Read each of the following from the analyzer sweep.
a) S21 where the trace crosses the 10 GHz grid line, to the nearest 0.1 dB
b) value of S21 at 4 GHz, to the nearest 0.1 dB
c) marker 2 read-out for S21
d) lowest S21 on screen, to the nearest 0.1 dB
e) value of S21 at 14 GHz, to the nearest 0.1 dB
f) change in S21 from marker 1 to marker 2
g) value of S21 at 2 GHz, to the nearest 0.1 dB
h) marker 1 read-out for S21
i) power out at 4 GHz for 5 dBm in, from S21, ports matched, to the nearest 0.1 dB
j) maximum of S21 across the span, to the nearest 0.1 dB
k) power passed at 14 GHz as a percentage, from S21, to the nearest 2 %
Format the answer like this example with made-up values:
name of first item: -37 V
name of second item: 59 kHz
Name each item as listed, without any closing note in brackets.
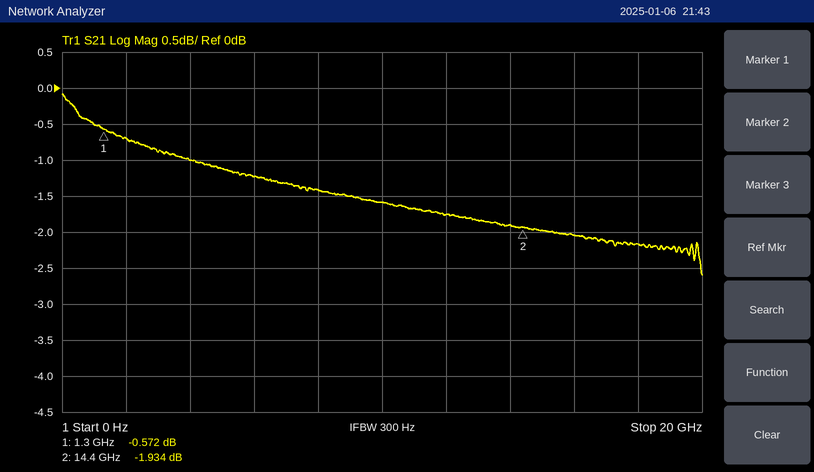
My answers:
S21 where the trace crosses the 10 GHz grid line, to the nearest 0.1 dB: -1.6 dB
value of S21 at 4 GHz, to the nearest 0.1 dB: -1.0 dB
marker 2 read-out for S21: -1.934 dB
lowest S21 on screen, to the nearest 0.1 dB: -2.6 dB
value of S21 at 14 GHz, to the nearest 0.1 dB: -1.9 dB
change in S21 from marker 1 to marker 2: -1.362 dB
value of S21 at 2 GHz, to the nearest 0.1 dB: -0.7 dB
marker 1 read-out for S21: -0.572 dB
power out at 4 GHz for 5 dBm in, from S21, ports matched, to the nearest 0.1 dB: 4.0 dBm
maximum of S21 across the span, to the nearest 0.1 dB: -0.1 dB
power passed at 14 GHz as a percentage, from S21, to the nearest 2 %: 64 %
